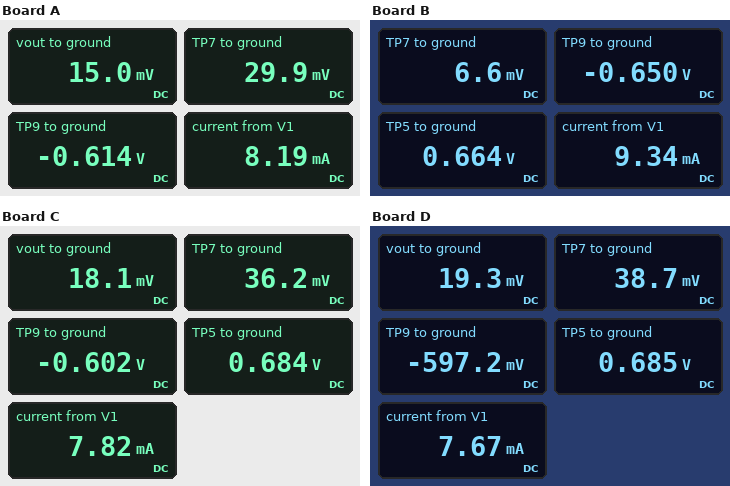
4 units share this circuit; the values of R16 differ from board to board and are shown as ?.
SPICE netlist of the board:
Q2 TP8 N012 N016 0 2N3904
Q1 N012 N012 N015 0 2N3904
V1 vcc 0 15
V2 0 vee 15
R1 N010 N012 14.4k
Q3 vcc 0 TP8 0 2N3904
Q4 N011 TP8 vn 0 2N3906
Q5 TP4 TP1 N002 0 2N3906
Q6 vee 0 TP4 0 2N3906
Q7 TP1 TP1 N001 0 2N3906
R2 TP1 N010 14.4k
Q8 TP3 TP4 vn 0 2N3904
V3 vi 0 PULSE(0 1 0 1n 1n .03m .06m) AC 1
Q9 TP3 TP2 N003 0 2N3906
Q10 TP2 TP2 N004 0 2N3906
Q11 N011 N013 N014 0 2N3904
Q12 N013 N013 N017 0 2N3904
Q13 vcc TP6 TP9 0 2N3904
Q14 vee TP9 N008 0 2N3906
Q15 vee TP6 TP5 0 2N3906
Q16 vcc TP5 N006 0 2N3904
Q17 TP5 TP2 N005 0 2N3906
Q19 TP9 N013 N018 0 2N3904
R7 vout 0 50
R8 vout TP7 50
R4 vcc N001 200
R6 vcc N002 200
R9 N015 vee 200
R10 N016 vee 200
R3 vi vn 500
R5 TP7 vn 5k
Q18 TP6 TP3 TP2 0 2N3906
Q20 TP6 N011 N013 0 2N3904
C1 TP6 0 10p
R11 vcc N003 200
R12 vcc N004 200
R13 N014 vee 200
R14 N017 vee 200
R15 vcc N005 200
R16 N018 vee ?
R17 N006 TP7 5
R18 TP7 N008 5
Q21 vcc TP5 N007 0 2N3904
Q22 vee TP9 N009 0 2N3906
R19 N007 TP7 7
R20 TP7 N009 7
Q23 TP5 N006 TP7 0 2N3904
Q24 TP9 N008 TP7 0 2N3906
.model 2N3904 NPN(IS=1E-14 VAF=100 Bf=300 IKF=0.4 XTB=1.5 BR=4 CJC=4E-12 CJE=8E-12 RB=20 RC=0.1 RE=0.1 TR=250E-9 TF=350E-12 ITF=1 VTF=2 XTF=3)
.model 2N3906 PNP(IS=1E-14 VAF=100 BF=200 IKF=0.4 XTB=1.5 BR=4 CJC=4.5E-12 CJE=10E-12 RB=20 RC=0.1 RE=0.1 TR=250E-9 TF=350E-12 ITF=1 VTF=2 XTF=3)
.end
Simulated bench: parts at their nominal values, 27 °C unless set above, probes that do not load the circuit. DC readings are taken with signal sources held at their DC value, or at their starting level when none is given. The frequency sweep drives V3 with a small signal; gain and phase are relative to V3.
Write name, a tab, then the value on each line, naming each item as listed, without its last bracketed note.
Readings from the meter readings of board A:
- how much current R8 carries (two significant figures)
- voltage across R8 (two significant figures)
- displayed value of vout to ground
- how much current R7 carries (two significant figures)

how much current R8 carries	300 µA
voltage across R8	15 mV
displayed value of vout to ground	15.0 mV
how much current R7 carries	300 µA
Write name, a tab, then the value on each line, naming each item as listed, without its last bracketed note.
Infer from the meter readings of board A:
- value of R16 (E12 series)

value of R16	270 Ω
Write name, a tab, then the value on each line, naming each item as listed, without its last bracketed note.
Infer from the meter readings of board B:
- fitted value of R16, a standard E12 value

fitted value of R16, a standard E12 value	120 Ω
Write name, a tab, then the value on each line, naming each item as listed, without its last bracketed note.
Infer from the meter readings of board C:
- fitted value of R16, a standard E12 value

fitted value of R16, a standard E12 value	390 Ω
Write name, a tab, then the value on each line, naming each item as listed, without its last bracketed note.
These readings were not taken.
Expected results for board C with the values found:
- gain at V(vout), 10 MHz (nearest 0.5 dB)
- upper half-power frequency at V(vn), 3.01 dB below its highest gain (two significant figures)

gain at V(vout), 10 MHz	-1.5 dB
upper half-power frequency at V(vn), 3.01 dB below its highest gain	2.0 GHz
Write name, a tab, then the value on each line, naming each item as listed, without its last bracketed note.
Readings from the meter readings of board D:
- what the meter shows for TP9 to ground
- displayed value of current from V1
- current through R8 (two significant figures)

what the meter shows for TP9 to ground	-597.2 mV
displayed value of current from V1	7.67 mA
current through R8	390 µA
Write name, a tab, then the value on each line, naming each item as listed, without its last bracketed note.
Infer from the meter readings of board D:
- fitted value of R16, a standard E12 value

fitted value of R16, a standard E12 value	470 Ω
